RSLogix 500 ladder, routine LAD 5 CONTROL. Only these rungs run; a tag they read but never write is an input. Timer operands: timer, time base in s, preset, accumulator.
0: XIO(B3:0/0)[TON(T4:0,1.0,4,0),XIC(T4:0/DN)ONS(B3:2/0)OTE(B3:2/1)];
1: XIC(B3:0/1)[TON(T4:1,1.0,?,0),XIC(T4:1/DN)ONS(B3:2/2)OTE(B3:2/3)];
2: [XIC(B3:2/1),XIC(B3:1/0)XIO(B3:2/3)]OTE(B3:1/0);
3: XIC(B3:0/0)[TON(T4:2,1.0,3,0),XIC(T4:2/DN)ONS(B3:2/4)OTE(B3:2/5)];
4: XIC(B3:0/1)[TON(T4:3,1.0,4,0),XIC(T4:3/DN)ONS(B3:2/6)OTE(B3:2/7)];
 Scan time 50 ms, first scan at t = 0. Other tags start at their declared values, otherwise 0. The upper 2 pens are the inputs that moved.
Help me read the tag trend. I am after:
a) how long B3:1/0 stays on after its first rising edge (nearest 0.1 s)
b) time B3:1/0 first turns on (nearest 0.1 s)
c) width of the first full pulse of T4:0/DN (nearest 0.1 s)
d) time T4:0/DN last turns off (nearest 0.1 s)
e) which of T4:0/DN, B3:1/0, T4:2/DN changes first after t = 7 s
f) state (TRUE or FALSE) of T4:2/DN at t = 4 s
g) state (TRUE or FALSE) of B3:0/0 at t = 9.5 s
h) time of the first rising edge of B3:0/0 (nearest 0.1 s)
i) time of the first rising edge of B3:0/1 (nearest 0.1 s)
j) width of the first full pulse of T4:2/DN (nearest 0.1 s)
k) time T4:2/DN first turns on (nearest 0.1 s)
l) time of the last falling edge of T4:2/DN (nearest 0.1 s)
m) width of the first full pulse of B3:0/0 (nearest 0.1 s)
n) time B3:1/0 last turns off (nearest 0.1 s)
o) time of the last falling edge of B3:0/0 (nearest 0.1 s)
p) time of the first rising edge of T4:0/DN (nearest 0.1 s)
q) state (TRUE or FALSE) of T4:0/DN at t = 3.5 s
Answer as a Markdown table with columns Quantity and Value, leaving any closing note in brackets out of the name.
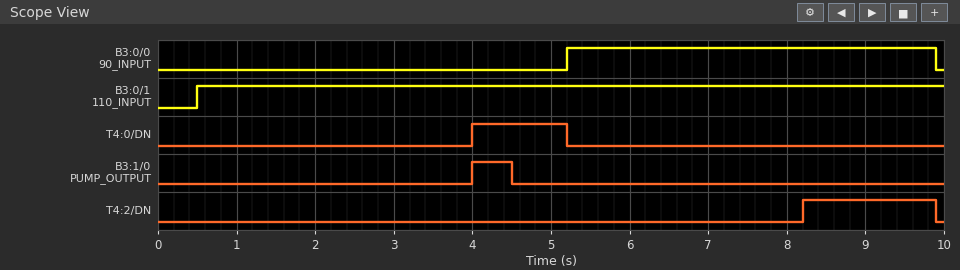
| Quantity | Value |
|---|---|
| how long B3:1/0 stays on after its first rising edge | 0.5 s |
| time B3:1/0 first turns on | 4.0 s |
| width of the first full pulse of T4:0/DN | 1.2 s |
| time T4:0/DN last turns off | 5.2 s |
| which of T4:0/DN, B3:1/0, T4:2/DN changes first after t = 7 s | T4:2/DN |
| state (TRUE or FALSE) of T4:2/DN at t = 4 s | FALSE |
| state (TRUE or FALSE) of B3:0/0 at t = 9.5 s | TRUE |
| time of the first rising edge of B3:0/0 | 5.2 s |
| time of the first rising edge of B3:0/1 | 0.5 s |
| width of the first full pulse of T4:2/DN | 1.7 s |
| time T4:2/DN first turns on | 8.2 s |
| time of the last falling edge of T4:2/DN | 9.9 s |
| width of the first full pulse of B3:0/0 | 4.7 s |
| time B3:1/0 last turns off | 4.5 s |
| time of the last falling edge of B3:0/0 | 9.9 s |
| time of the first rising edge of T4:0/DN | 4.0 s |
| state (TRUE or FALSE) of T4:0/DN at t = 3.5 s | FALSE |
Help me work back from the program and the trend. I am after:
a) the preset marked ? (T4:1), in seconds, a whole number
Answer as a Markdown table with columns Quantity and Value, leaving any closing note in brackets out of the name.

| Quantity | Value |
|---|---|
| the preset marked ? (T4:1), in seconds, a whole number | 4 s |
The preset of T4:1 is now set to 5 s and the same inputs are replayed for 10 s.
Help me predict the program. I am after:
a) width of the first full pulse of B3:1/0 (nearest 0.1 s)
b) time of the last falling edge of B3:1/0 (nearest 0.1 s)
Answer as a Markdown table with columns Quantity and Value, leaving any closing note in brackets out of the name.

| Quantity | Value |
|---|---|
| width of the first full pulse of B3:1/0 | 1.5 s |
| time of the last falling edge of B3:1/0 | 5.5 s |
